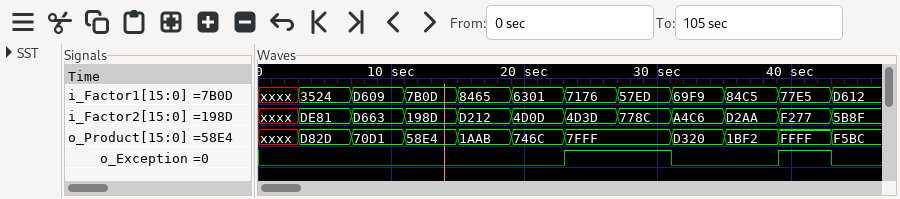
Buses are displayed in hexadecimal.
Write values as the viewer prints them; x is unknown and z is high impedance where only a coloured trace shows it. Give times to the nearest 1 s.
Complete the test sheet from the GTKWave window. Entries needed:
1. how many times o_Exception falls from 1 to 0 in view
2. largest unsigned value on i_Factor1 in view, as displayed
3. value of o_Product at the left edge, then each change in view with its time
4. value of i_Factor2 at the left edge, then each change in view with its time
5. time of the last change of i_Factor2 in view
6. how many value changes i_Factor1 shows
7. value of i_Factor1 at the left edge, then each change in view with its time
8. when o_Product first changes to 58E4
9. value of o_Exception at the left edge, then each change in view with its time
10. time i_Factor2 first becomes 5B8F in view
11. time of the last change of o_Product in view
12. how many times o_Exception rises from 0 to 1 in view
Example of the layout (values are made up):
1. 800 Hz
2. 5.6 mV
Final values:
1. 2
2. D612
3. xxxx, D82D at 3 s, 70D1 at 7 s, 58E4 at 11 s, 1AAB at 15 s, 746C at 19 s, 7FFF at 23 s, D320 at 31 s, 1BF2 at 35 s, FFFF at 39 s, F5BC at 43 s
4. xxxx, DE81 at 3 s, D663 at 7 s, 198D at 11 s, D212 at 15 s, 4D0D at 19 s, 4D3D at 23 s, 778C at 27 s, A4C6 at 31 s, D2AA at 35 s, F277 at 39 s, 5B8F at 43 s
5. 43 s
6. 11
7. xxxx, 3524 at 3 s, D609 at 7 s, 7B0D at 11 s, 8465 at 15 s, 6301 at 19 s, 7176 at 23 s, 57ED at 27 s, 69F9 at 31 s, 84C5 at 35 s, 77E5 at 39 s, D612 at 43 s
8. 11 s
9. 0, 1 at 23 s, 0 at 31 s, 1 at 39 s, 0 at 43 s
10. 43 s
11. 43 s
12. 2
